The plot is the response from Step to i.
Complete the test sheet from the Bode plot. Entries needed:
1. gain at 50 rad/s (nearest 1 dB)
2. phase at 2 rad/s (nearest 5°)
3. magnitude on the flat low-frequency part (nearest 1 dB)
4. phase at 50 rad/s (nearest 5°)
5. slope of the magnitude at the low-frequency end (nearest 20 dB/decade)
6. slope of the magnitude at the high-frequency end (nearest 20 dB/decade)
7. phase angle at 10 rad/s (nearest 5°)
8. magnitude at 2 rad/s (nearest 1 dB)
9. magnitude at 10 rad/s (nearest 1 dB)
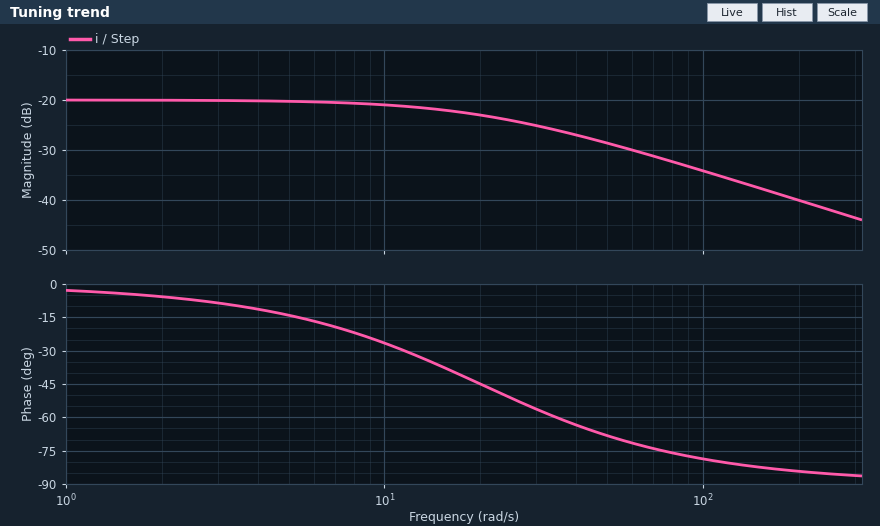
-29 dB
-5°
-20 dB
-70°
0 dB/decade
-20 dB/decade
-25°
-20 dB
-21 dB
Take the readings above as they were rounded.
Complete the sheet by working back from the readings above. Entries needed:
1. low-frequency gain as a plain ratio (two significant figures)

0.10
